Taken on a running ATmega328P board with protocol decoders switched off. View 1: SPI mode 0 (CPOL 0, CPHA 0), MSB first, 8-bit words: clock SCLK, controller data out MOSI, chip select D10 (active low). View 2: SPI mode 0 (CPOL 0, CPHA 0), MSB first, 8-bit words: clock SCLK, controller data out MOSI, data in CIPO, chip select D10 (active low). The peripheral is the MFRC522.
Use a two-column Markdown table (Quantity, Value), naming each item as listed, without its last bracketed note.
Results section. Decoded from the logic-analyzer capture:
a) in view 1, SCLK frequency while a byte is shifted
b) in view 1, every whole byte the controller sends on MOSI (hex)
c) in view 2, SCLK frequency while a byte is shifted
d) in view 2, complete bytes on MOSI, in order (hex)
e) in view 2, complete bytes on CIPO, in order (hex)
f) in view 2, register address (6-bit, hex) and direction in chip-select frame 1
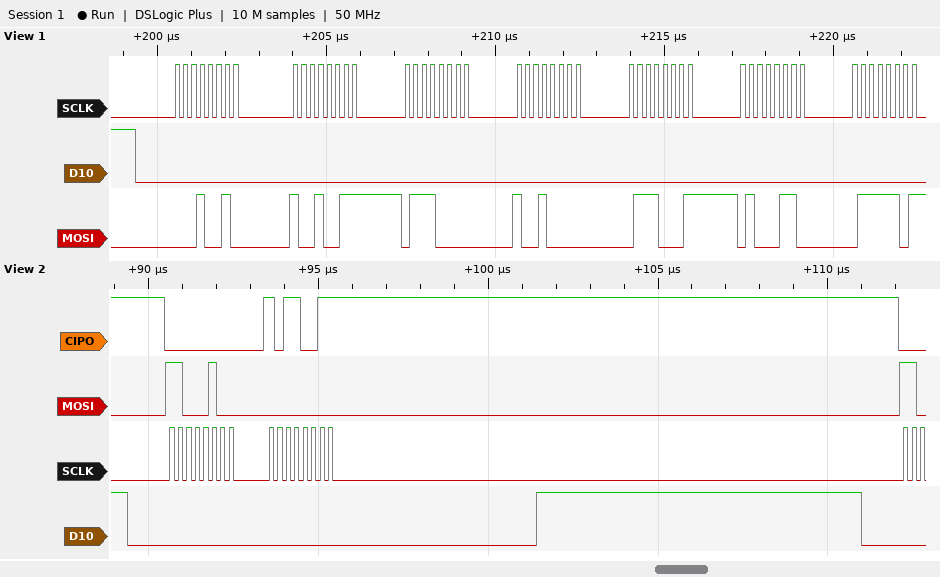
| Quantity | Value |
|---|---|
| in view 1, SCLK frequency while a byte is shifted | 4 MHz |
| in view 1, every whole byte the controller sends on MOSI | 0x12 0x93 0x70 0x90 0x71 0x46 0x7D |
| in view 2, SCLK frequency while a byte is shifted | 4 MHz |
| in view 2, complete bytes on MOSI, in order | C4 00 |
| in view 2, complete bytes on CIPO, in order | 00 B3 |
| in view 2, register address (6-bit, hex) and direction in chip-select frame 1 | 0x22 read |
